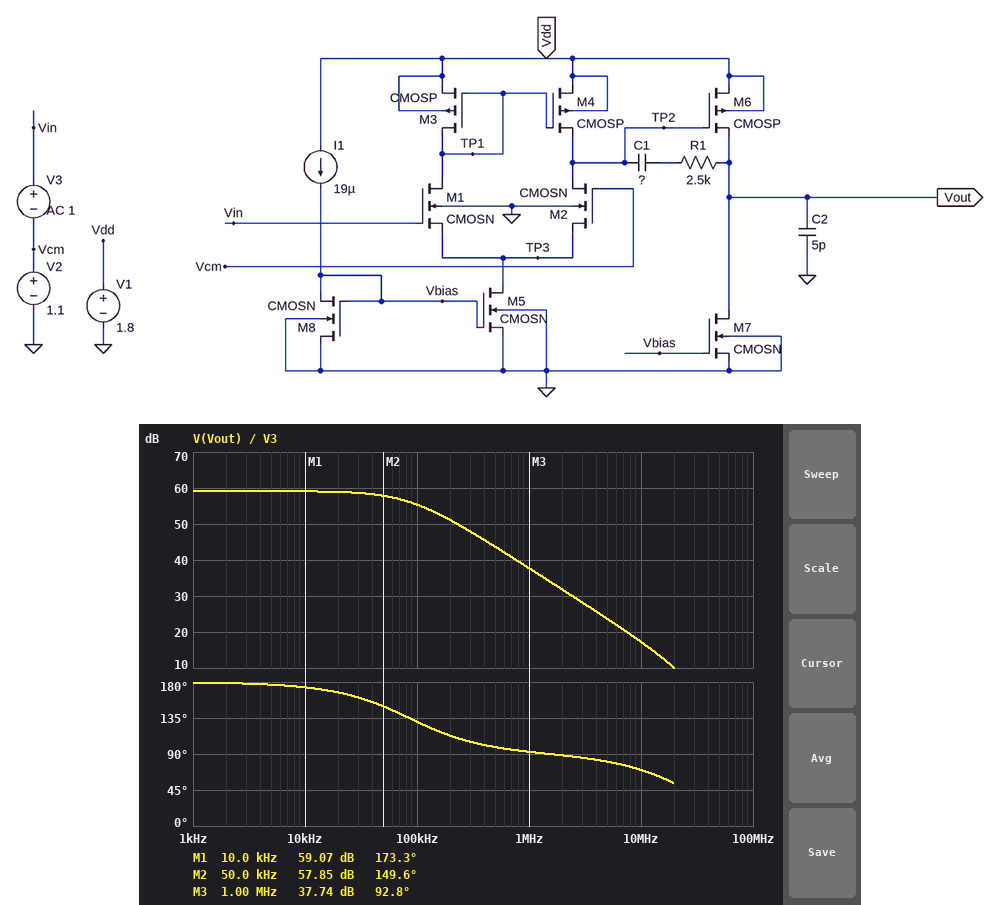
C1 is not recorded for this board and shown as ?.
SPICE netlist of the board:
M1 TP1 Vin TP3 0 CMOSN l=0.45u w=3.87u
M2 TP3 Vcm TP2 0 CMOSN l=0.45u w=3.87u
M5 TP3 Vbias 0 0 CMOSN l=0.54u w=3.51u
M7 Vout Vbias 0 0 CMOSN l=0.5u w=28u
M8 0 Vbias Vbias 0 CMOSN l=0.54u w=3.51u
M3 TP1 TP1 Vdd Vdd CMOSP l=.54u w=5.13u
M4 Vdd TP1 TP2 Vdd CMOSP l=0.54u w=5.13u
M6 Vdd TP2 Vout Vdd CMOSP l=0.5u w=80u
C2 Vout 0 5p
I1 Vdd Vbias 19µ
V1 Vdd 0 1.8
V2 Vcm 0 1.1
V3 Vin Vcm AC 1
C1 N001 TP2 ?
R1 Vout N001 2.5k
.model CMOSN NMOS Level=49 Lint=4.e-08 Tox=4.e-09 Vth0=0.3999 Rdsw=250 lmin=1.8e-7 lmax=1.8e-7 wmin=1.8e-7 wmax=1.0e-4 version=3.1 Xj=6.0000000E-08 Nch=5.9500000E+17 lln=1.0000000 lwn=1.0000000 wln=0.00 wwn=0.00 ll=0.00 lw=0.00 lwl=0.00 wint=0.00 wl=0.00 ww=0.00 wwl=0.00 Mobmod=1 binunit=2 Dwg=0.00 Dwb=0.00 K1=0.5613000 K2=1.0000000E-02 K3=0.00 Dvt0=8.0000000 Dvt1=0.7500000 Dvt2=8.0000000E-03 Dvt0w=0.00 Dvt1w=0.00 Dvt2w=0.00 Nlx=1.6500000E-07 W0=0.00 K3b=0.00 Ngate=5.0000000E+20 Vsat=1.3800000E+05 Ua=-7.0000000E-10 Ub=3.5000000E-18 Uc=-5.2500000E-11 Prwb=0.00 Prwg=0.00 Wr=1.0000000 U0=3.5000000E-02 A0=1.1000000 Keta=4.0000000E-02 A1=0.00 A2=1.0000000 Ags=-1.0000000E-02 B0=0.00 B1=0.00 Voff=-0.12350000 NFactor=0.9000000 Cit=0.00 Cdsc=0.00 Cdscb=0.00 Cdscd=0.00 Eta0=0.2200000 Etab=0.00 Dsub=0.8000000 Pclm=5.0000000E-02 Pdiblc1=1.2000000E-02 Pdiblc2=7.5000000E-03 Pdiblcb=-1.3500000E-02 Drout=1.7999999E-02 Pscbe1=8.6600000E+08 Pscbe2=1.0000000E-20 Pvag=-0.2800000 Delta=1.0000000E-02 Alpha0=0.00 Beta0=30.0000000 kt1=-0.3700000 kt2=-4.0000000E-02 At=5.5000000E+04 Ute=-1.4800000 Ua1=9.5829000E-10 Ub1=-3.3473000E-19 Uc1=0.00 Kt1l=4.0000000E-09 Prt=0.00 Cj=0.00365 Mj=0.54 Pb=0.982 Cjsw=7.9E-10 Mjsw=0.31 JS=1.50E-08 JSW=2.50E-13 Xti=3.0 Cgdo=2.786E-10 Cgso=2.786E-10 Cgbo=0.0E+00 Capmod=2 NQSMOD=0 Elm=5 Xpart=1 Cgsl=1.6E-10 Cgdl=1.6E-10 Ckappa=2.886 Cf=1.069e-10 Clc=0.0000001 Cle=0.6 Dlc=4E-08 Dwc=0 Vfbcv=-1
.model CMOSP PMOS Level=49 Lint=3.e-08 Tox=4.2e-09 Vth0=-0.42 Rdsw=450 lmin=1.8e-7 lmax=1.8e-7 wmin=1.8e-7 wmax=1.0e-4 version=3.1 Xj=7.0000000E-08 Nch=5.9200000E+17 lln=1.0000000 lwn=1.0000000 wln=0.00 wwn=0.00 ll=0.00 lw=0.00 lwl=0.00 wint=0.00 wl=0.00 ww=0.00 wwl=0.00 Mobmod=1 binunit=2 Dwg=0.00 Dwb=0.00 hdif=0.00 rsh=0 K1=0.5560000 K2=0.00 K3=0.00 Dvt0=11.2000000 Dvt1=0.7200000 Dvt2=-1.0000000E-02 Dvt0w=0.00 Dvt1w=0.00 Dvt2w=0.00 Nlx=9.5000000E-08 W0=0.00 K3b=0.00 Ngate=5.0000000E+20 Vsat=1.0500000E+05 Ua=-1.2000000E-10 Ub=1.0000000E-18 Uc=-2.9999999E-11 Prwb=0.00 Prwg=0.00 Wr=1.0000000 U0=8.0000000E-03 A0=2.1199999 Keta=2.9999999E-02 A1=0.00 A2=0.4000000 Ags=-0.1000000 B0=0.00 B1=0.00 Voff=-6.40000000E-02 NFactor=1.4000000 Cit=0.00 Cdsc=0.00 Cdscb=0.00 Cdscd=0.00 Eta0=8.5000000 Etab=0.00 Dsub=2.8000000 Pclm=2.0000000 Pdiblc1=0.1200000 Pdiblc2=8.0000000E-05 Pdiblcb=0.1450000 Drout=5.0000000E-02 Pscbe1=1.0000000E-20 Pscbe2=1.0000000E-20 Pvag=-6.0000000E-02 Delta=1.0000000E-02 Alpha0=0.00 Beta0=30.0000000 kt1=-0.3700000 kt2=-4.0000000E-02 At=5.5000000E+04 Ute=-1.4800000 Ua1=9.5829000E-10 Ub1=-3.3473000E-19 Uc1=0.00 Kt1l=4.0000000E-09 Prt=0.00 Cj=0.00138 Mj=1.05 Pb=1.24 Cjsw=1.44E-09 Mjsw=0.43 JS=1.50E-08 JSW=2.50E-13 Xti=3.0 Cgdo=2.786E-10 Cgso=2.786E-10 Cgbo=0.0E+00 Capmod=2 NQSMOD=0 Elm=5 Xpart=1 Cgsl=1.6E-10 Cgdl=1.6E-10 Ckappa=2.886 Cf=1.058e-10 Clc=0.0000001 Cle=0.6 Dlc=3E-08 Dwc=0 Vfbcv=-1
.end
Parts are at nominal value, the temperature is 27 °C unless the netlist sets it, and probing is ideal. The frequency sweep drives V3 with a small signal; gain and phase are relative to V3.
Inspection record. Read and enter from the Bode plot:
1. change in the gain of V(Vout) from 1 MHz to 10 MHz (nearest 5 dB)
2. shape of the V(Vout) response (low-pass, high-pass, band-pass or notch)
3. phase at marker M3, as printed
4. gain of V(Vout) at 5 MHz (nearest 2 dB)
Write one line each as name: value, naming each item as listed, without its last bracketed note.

change in the gain of V(Vout) from 1 MHz to 10 MHz: -20 dB
shape of the V(Vout) response: low-pass
phase at marker M3, as printed: 92.8 deg
gain of V(Vout) at 5 MHz: 24 dB
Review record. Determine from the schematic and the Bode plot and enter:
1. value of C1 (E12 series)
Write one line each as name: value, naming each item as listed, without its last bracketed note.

value of C1: 220 fF
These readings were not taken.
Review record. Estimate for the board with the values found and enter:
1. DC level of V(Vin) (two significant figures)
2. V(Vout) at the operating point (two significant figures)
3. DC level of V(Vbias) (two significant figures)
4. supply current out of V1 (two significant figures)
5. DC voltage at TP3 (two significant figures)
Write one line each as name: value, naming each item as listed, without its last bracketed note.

DC level of V(Vin): 1.1 V
V(Vout) at the operating point: 930 mV
DC level of V(Vbias): 610 mV
supply current out of V1: 200 µA
DC voltage at TP3: 430 mV
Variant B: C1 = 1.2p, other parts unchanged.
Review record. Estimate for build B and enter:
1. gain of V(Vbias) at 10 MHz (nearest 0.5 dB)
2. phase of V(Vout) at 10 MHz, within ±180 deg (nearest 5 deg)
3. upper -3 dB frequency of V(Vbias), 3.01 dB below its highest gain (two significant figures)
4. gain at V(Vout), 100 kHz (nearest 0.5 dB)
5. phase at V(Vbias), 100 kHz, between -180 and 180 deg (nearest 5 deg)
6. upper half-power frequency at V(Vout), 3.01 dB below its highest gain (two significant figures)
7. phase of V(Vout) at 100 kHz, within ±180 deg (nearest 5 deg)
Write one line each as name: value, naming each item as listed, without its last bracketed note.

gain of V(Vbias) at 10 MHz: -43.0 dB
phase of V(Vout) at 10 MHz, within ±180 deg: 85 deg
upper -3 dB frequency of V(Vbias), 3.01 dB below its highest gain: 1.5 GHz
gain at V(Vout), 100 kHz: 44.5 dB
phase at V(Vbias), 100 kHz, between -180 and 180 deg: -170 deg
upper half-power frequency at V(Vout), 3.01 dB below its highest gain: 19 kHz
phase of V(Vout) at 100 kHz, within ±180 deg: 100 deg
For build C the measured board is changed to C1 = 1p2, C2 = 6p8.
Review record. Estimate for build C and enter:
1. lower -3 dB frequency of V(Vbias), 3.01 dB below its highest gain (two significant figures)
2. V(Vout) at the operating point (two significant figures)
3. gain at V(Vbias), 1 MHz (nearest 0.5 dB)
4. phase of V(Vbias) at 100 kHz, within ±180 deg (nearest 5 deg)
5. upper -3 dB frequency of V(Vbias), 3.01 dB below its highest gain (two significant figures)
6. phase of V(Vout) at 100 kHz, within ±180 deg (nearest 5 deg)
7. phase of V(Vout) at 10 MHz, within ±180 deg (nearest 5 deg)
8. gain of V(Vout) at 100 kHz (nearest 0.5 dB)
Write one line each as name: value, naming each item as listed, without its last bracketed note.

lower -3 dB frequency of V(Vbias), 3.01 dB below its highest gain: 19 kHz
V(Vout) at the operating point: 930 mV
gain at V(Vbias), 1 MHz: -43.0 dB
phase of V(Vbias) at 100 kHz, within ±180 deg: -170 deg
upper -3 dB frequency of V(Vbias), 3.01 dB below its highest gain: 1.5 GHz
phase of V(Vout) at 100 kHz, within ±180 deg: 100 deg
phase of V(Vout) at 10 MHz, within ±180 deg: 80 deg
gain of V(Vout) at 100 kHz: 44.5 dB
